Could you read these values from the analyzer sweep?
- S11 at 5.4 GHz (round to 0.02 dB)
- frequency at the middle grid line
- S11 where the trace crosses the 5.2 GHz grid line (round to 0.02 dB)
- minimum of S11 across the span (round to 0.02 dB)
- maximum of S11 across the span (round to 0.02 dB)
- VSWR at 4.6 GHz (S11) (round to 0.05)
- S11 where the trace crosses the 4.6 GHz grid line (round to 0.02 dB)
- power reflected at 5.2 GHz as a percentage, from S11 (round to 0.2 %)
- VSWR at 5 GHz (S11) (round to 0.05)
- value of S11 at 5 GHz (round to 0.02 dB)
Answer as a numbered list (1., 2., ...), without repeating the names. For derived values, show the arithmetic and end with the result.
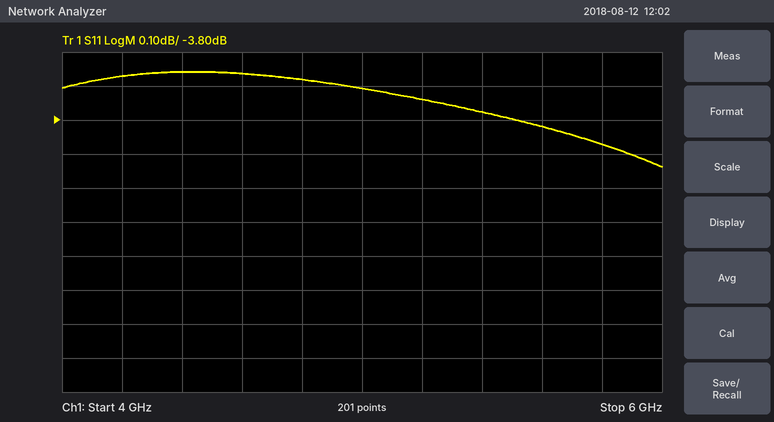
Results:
1. -3.78 dB
2. 5 GHz
3. -3.74 dB
4. -3.94 dB
5. -3.66 dB
6. |Γ| = 10^(-3.66/20) = 0.6561; VSWR = (1 + 0.6561)/(1 − 0.6561) ≈ 4.82, so 4.80 to the nearest 0.05
7. -3.66 dB
8. 10^(-3.74/10) ≈ 42.3 %, so 42.2 % to the nearest 0.2 %
9. |Γ| = 10^(-3.7/20) = 0.6531; VSWR = (1 + 0.6531)/(1 − 0.6531) ≈ 4.77, so 4.75 to the nearest 0.05
10. -3.70 dB
